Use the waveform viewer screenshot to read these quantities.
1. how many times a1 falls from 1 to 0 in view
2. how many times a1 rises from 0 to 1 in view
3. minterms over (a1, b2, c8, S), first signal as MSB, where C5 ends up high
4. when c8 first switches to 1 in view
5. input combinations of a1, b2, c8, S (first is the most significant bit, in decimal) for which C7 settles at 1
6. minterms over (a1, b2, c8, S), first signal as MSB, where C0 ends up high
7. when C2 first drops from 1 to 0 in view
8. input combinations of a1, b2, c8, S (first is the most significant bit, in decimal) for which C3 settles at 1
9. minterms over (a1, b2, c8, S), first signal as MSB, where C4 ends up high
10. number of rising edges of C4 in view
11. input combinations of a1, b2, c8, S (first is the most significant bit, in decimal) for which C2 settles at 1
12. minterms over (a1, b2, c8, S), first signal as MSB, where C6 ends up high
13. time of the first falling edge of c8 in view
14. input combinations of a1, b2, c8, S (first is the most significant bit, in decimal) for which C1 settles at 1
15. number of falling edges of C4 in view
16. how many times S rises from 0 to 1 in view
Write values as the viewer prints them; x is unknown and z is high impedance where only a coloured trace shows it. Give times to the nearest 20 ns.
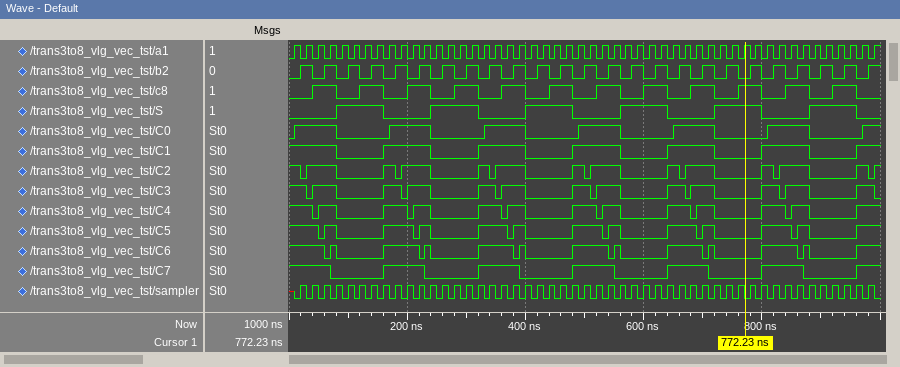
49
50
0, 2, 4, 6, 8, 12, 14
40 ns
0, 2, 4, 6, 8, 10, 12
2, 4, 6, 8, 10, 12, 14
20 ns
0, 2, 4, 6, 8, 10, 14
0, 4, 6, 8, 10, 12, 14
12
0, 2, 6, 8, 10, 12, 14
0, 2, 4, 8, 10, 12, 14
80 ns
0, 2, 4, 6, 8, 10, 12, 14
12
6
